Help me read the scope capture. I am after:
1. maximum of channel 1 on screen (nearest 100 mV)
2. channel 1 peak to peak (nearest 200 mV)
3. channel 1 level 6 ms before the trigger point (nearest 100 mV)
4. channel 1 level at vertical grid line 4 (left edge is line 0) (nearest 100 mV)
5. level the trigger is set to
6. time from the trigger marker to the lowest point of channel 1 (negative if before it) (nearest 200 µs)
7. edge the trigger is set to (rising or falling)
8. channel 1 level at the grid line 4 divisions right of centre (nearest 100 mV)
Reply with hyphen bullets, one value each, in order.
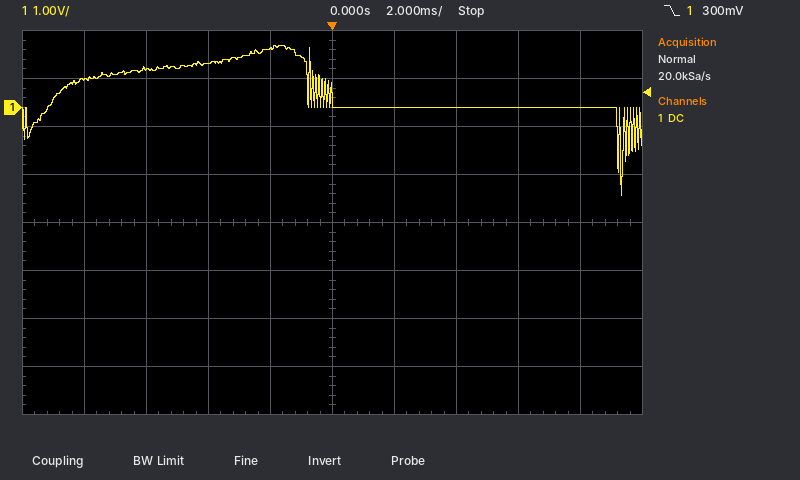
- 1.3 V
- 3.2 V
- 800 mV
- 1.2 V
- 300 mV
- +9.4 ms
- falling
- 0.0 V
